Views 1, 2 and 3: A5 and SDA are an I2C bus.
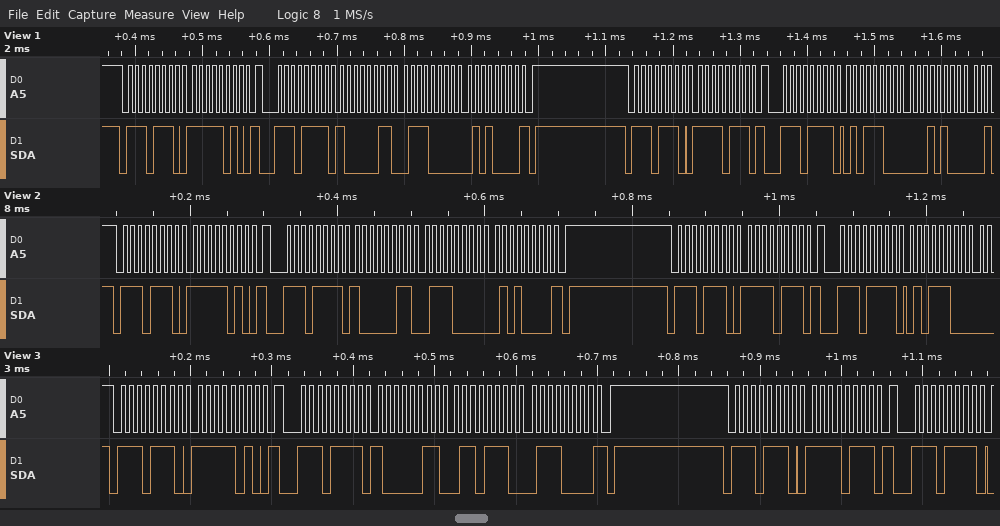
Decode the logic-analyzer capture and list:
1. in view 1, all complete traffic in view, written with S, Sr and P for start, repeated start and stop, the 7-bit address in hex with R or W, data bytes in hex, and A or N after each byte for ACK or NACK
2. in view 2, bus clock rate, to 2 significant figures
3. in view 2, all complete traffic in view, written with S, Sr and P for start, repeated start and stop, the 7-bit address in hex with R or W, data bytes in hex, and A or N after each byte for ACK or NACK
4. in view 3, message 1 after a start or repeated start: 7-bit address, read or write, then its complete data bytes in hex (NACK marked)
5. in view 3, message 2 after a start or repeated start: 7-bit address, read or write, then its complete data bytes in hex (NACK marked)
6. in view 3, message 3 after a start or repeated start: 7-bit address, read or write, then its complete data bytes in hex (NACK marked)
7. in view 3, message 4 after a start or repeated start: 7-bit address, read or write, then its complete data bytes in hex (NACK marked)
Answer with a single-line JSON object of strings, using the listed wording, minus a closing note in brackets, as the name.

{"in view 1, all complete traffic in view, written with S, Sr and P for start, repeated start and stop, the 7-bit address in hex with R or W, data bytes in hex, and A or N after each byte for ACK or NACK": "S 77W A FA A Sr 77R A 83 A 70 A 50 N P S 77W A F7 A Sr 77R A 5C A 14 A", "in view 2, bus clock rate, to 2 significant figures": "100 kHz", "in view 2, all complete traffic in view, written with S, Sr and P for start, repeated start and stop, the 7-bit address in hex with R or W, data bytes in hex, and A or N after each byte for ACK or NACK": "S 77W A FA A Sr 77R A 83 A 70 A 50 N P S 77W A F7 A Sr 77R A 5C A", "in view 3, message 1 after a start or repeated start: 7-bit address, read or write, then its complete data bytes in hex": "0x77 write: FA", "in view 3, message 2 after a start or repeated start: 7-bit address, read or write, then its complete data bytes in hex": "0x77 read: 83 6E 70 NACK", "in view 3, message 3 after a start or repeated start: 7-bit address, read or write, then its complete data bytes in hex": "0x77 write: F7", "in view 3, message 4 after a start or repeated start: 7-bit address, read or write, then its complete data bytes in hex": "0x77 read"}
